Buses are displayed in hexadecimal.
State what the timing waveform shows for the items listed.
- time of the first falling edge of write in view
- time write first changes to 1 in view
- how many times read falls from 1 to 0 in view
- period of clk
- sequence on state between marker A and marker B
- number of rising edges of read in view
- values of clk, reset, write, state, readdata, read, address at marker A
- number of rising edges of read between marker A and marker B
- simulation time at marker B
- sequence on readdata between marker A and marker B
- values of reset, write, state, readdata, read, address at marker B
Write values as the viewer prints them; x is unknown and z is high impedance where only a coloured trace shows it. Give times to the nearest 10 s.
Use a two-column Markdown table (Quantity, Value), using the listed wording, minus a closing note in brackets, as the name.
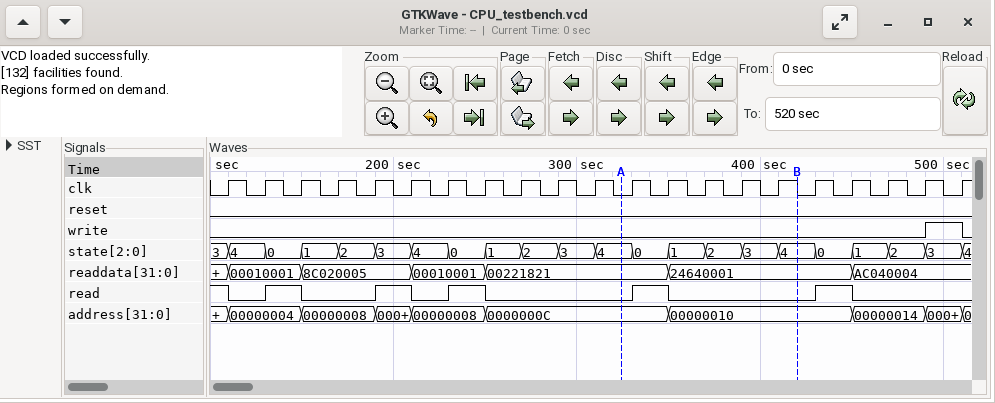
| Quantity | Value |
|---|---|
| time of the first falling edge of write in view | 510 s |
| time write first changes to 1 in view | 490 s |
| how many times read falls from 1 to 0 in view | 6 |
| period of clk | 20 s |
| sequence on state between marker A and marker B | 4, 0, 1, 2, 3, 4 |
| number of rising edges of read in view | 5 |
| values of clk, reset, write, state, readdata, read, address at marker A | clk=0, reset=0, write=0, state=4, readdata=00221821, read=0, address=0000000C |
| number of rising edges of read between marker A and marker B | 1 |
| simulation time at marker B | 420 s |
| sequence on readdata between marker A and marker B | 00221821, 24640001 |
| values of reset, write, state, readdata, read, address at marker B | reset=0, write=0, state=4, readdata=24640001, read=0, address=00000010 |
